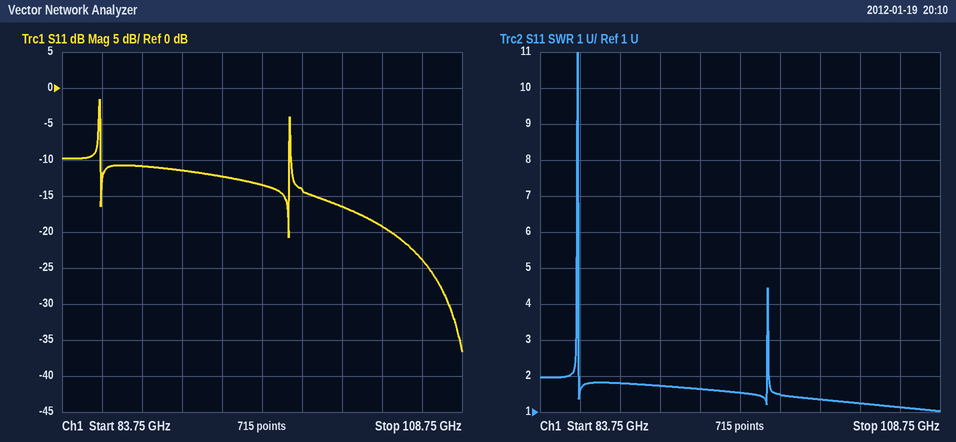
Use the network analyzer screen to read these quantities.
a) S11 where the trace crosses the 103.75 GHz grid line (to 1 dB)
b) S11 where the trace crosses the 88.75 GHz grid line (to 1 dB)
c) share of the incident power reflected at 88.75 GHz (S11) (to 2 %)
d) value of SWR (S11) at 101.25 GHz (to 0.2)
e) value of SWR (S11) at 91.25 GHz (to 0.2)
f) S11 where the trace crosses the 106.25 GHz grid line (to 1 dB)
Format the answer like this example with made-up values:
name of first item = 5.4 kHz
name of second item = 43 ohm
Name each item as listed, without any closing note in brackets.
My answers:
S11 where the trace crosses the 103.75 GHz grid line = -19 dB
S11 where the trace crosses the 88.75 GHz grid line = -11 dB
share of the incident power reflected at 88.75 GHz (S11) = 8 %
value of SWR (S11) at 101.25 GHz = 1.4
value of SWR (S11) at 91.25 GHz = 1.8
S11 where the trace crosses the 106.25 GHz grid line = -24 dB
